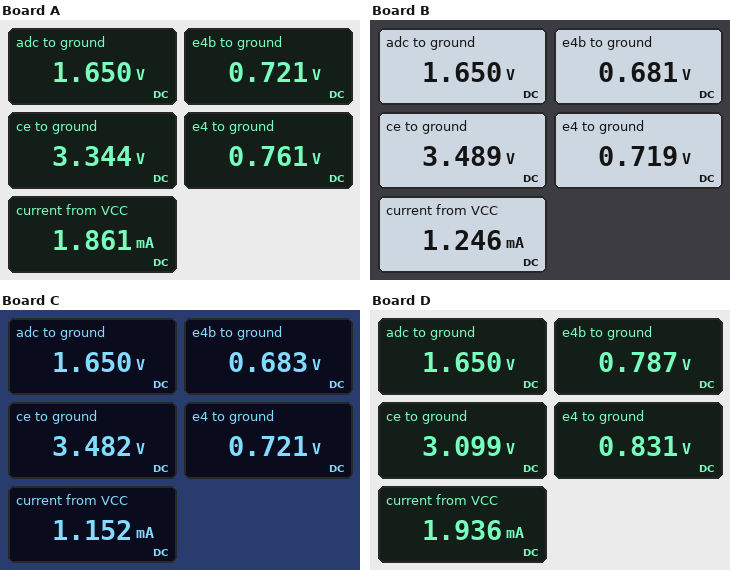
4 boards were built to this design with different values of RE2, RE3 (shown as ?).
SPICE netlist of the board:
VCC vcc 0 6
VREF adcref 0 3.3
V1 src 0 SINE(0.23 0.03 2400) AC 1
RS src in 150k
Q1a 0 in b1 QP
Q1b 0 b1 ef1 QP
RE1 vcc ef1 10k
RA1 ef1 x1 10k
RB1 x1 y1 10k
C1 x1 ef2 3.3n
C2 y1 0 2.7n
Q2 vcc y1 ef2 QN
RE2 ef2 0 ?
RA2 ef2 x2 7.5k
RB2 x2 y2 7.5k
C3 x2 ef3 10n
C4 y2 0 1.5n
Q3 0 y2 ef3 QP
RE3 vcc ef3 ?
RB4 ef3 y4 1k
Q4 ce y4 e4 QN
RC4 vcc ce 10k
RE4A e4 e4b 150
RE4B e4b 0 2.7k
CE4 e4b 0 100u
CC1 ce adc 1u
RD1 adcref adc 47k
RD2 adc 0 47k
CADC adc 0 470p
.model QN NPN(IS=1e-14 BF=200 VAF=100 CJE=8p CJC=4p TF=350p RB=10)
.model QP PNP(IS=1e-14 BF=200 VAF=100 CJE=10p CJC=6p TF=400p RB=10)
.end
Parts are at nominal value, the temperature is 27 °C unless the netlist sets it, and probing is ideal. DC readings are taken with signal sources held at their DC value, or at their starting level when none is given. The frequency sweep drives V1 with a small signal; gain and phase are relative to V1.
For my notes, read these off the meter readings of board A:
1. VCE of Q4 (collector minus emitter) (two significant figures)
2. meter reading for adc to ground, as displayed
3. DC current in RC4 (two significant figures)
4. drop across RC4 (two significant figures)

2.6 V
1.650 V
270 µA
2.7 V
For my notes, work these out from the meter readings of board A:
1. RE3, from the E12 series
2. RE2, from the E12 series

6.8 kΩ
1.5 kΩ
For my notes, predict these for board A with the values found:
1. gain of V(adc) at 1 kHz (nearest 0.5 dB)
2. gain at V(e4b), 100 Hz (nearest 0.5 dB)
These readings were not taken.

27.5 dB
-25.0 dB
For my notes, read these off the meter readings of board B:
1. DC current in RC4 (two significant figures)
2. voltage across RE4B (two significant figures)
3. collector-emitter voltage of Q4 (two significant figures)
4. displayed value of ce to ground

250 µA
680 mV
2.8 V
3.489 V
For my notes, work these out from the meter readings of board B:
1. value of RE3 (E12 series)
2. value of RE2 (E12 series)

22 kΩ
2.2 kΩ
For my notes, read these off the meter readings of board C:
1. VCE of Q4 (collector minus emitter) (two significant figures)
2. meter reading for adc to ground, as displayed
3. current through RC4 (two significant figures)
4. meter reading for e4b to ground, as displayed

2.8 V
1.650 V
250 µA
0.683 V
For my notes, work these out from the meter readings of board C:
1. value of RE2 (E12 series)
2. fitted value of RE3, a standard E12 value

2.7 kΩ
27 kΩ
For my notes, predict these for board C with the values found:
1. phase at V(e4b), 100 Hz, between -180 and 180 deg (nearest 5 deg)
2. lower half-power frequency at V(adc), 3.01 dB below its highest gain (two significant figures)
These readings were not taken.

-90 deg
8.9 Hz
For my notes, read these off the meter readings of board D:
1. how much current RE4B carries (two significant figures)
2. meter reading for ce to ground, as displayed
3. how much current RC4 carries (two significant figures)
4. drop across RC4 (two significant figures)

290 µA
3.099 V
290 µA
2.9 V
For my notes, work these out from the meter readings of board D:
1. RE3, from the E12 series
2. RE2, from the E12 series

4.7 kΩ
3.3 kΩ
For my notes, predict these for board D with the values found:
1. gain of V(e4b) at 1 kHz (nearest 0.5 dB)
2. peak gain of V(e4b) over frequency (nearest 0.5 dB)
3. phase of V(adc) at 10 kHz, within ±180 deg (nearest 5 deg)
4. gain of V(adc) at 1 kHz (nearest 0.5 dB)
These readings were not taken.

-44.5 dB
-1.5 dB
-105 deg
28.0 dB
